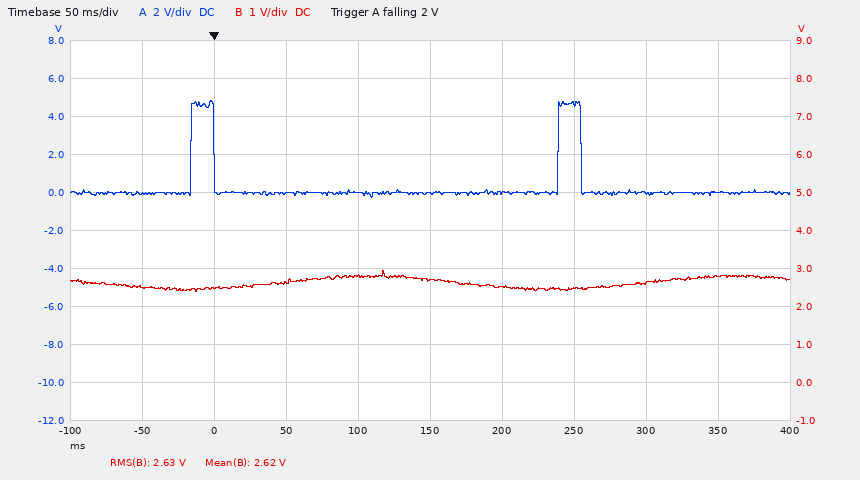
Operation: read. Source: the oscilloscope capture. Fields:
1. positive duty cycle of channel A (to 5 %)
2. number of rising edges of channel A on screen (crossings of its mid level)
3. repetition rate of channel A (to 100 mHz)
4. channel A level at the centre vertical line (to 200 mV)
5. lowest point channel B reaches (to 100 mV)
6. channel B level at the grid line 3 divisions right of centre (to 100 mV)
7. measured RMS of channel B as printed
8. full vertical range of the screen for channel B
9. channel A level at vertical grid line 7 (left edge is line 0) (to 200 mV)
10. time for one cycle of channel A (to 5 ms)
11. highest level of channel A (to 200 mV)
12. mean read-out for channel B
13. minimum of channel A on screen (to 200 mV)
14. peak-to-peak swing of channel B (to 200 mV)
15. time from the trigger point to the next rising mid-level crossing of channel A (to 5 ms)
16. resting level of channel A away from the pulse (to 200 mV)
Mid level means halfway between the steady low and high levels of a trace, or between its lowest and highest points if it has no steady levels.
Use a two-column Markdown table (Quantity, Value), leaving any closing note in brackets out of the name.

| Quantity | Value |
|---|---|
| positive duty cycle of channel A | 5 % |
| number of rising edges of channel A on screen | 2 |
| repetition rate of channel A | 3.9 Hz |
| channel A level at the centre vertical line | 0.0 V |
| lowest point channel B reaches | 2.4 V |
| channel B level at the grid line 3 divisions right of centre | 2.6 V |
| measured RMS of channel B as printed | 2.63 V |
| full vertical range of the screen for channel B | 10 V |
| channel A level at vertical grid line 7 (left edge is line 0) | 4.6 V |
| time for one cycle of channel A | 255 ms |
| highest level of channel A | 4.8 V |
| mean read-out for channel B | 2.62 V |
| minimum of channel A on screen | -200 mV |
| peak-to-peak swing of channel B | 600 mV |
| time from the trigger point to the next rising mid-level crossing of channel A | 240 ms |
| resting level of channel A away from the pulse | 0.0 V |
